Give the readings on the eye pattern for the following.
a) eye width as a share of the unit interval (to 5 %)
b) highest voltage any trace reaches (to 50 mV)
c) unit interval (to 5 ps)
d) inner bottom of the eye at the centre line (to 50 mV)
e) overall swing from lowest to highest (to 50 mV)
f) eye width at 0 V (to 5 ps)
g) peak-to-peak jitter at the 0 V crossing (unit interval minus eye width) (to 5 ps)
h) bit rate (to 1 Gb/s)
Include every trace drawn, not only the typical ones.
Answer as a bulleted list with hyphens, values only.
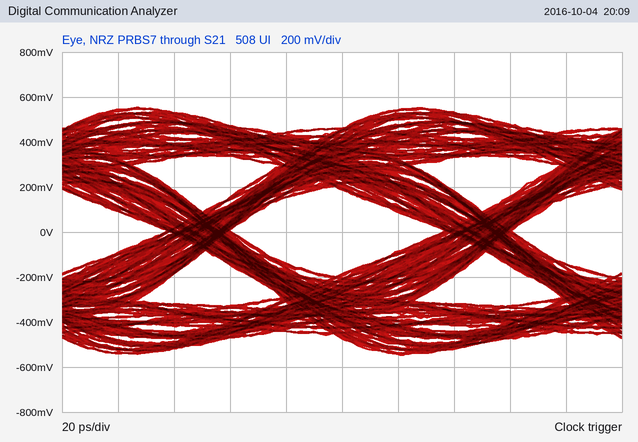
- 75 %
- 550 mV
- 100 ps
- -200 mV
- 1.10 V
- 75 ps
- 25 ps
- 10 Gb/s
